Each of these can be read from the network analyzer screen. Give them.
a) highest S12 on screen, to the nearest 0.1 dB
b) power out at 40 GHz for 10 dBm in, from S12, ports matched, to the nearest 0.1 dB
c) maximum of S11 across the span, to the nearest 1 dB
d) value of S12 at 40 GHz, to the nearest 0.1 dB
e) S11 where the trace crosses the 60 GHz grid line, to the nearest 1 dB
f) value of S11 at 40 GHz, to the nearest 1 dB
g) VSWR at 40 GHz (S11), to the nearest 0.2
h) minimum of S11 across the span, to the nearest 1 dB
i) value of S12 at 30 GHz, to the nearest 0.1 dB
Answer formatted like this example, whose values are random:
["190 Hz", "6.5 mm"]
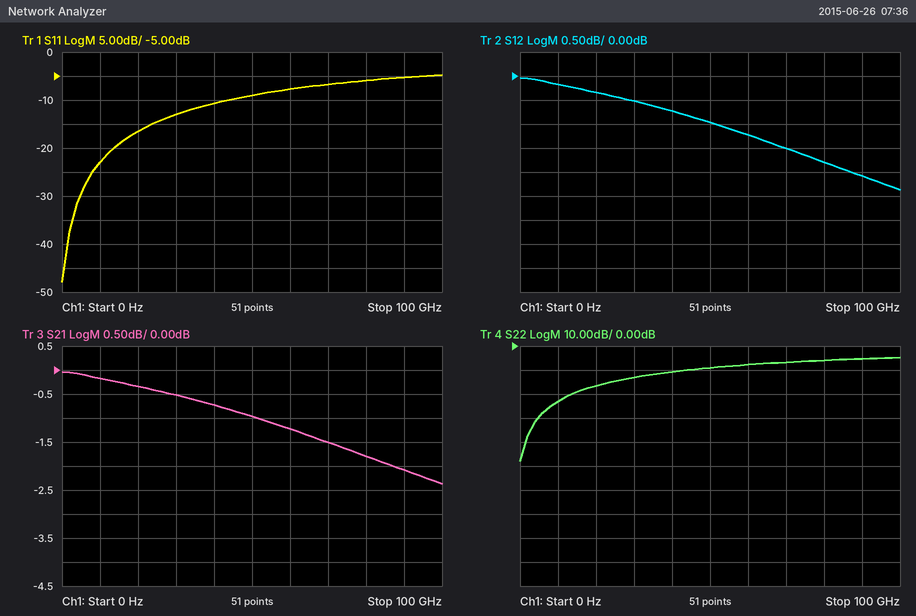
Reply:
["0.0 dB", "9.3 dBm", "-5 dB", "-0.7 dB", "-8 dB", "-11 dB", "1.8", "-48 dB", "-0.5 dB"]
